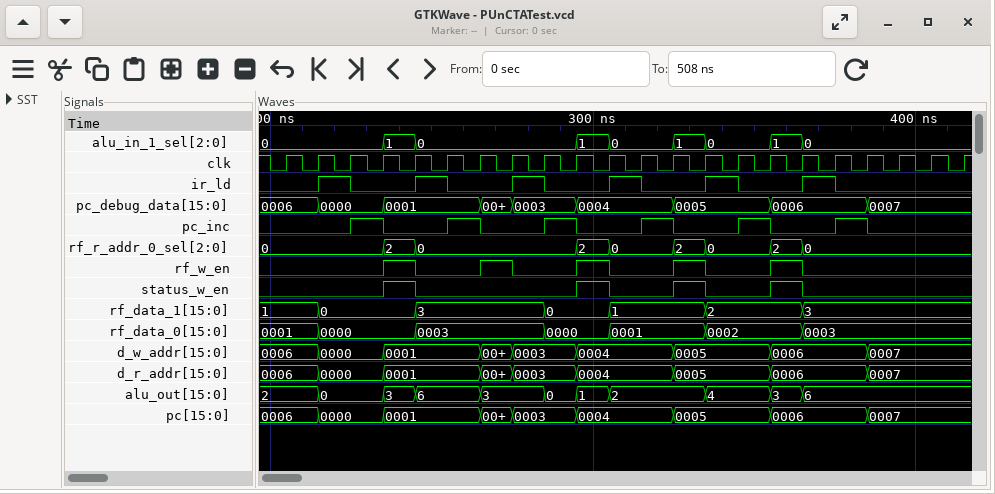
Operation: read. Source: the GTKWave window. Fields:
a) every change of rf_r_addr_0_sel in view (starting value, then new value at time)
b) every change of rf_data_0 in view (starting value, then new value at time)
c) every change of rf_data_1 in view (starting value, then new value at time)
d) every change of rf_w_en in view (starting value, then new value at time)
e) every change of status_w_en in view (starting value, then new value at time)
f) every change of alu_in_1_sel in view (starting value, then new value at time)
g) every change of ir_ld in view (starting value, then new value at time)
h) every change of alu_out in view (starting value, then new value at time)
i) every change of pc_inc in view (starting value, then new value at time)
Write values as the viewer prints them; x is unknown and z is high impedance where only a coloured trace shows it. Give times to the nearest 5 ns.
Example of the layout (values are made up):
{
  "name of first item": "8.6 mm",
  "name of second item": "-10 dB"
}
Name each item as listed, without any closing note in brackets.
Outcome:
{
  "every change of rf_r_addr_0_sel in view": "0, 2 at 235 ns, 0 at 245 ns, 2 at 295 ns, 0 at 305 ns, 2 at 325 ns, 0 at 335 ns, 2 at 355 ns, 0 at 365 ns",
  "every change of rf_data_0 in view": "0001, 0000 at 215 ns, 0003 at 245 ns, 0000 at 285 ns, 0001 at 305 ns, 0002 at 335 ns, 0003 at 365 ns",
  "every change of rf_data_1 in view": "1, 0 at 215 ns, 3 at 245 ns, 0 at 285 ns, 1 at 305 ns, 2 at 335 ns, 3 at 365 ns",
  "every change of rf_w_en in view": "0, 1 at 235 ns, 0 at 245 ns, 1 at 265 ns, 0 at 275 ns, 1 at 295 ns, 0 at 305 ns, 1 at 325 ns, 0 at 335 ns, 1 at 355 ns, 0 at 365 ns",
  "every change of status_w_en in view": "0, 1 at 235 ns, 0 at 245 ns, 1 at 295 ns, 0 at 305 ns, 1 at 325 ns, 0 at 335 ns, 1 at 355 ns, 0 at 365 ns",
  "every change of alu_in_1_sel in view": "0, 1 at 235 ns, 0 at 245 ns, 1 at 295 ns, 0 at 305 ns, 1 at 325 ns, 0 at 335 ns, 1 at 355 ns, 0 at 365 ns",
  "every change of ir_ld in view": "0, 1 at 215 ns, 0 at 225 ns, 1 at 245 ns, 0 at 255 ns, 1 at 275 ns, 0 at 285 ns, 1 at 305 ns, 0 at 315 ns, 1 at 335 ns, 0 at 345 ns, 1 at 365 ns, 0 at 375 ns",
  "every change of alu_out in view": "2, 0 at 215 ns, 3 at 235 ns, 6 at 245 ns, 3 at 265 ns, 0 at 285 ns, 1 at 295 ns, 2 at 305 ns, 4 at 335 ns, 3 at 355 ns, 6 at 365 ns",
  "every change of pc_inc in view": "0, 1 at 225 ns, 0 at 235 ns, 1 at 255 ns, 0 at 265 ns, 1 at 285 ns, 0 at 295 ns, 1 at 315 ns, 0 at 325 ns, 1 at 345 ns, 0 at 355 ns, 1 at 375 ns, 0 at 385 ns"
}
